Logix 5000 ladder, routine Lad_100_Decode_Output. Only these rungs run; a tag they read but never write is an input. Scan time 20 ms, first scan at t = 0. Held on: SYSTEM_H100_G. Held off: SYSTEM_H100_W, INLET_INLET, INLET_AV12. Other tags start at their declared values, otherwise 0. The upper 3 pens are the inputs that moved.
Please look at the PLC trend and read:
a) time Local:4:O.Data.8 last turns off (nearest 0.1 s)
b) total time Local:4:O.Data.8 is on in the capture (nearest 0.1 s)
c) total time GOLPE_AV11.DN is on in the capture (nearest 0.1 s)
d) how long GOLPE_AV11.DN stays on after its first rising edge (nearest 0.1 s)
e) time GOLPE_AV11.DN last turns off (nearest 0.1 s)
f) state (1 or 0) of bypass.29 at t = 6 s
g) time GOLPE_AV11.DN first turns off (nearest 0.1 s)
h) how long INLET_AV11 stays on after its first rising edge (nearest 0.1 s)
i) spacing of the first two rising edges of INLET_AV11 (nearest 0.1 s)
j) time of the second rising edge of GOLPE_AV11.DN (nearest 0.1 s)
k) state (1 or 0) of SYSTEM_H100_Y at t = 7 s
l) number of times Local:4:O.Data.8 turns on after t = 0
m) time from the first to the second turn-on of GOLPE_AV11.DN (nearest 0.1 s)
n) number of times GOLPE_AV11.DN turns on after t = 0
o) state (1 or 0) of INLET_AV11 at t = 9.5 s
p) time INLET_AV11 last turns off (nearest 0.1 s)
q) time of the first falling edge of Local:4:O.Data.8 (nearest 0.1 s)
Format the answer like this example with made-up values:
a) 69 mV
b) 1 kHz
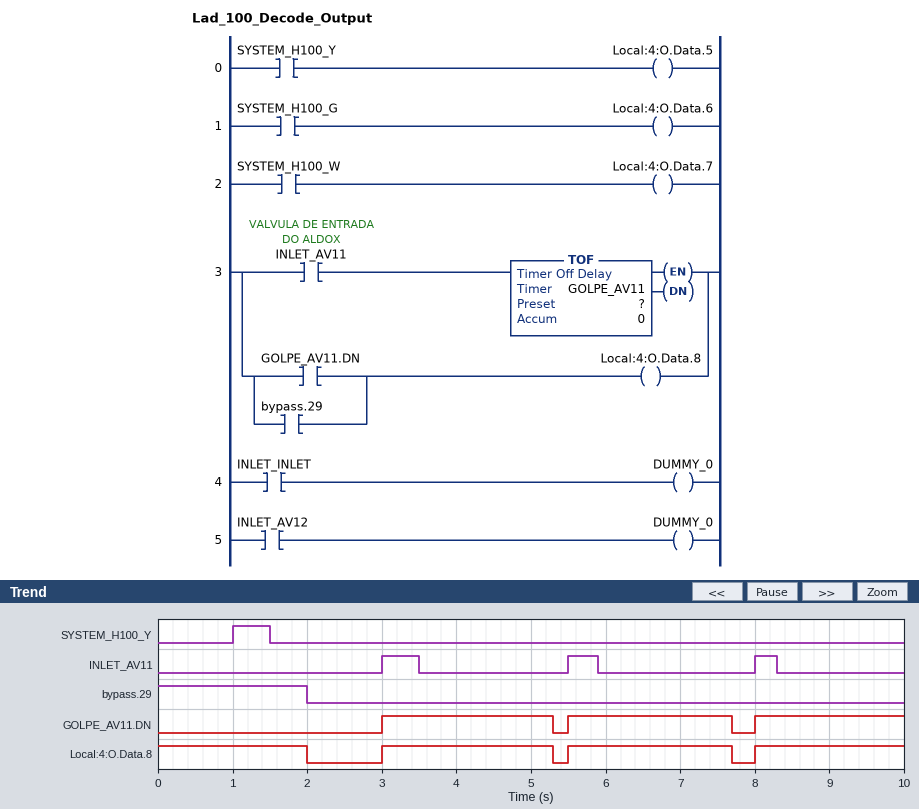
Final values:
a) 7.7 s
b) 8.5 s
c) 6.5 s
d) 2.3 s
e) 7.7 s
f) 0
g) 5.3 s
h) 0.5 s
i) 2.5 s
j) 5.5 s
k) 0
l) 3
m) 2.5 s
n) 3
o) 0
p) 8.3 s
q) 2.0 s
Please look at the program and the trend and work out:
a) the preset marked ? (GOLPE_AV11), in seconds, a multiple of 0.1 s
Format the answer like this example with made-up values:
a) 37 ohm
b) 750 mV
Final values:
a) 1.8 s
